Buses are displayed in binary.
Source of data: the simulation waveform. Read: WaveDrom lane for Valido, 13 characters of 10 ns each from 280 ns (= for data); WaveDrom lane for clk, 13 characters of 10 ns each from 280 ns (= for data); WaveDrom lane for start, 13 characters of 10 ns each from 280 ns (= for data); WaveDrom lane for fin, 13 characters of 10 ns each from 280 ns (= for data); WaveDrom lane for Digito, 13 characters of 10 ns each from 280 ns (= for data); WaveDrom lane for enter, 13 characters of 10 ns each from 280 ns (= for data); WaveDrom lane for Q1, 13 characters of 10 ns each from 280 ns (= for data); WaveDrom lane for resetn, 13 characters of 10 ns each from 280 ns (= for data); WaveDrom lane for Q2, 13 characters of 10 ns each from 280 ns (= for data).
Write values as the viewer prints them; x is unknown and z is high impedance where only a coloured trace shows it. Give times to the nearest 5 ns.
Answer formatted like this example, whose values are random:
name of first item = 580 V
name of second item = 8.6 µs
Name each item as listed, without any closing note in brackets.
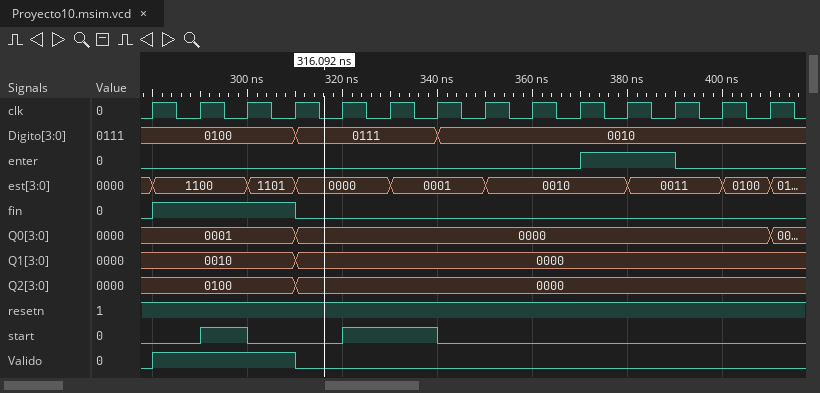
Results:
WaveDrom lane for Valido, 13 characters of 10 ns each from 280 ns = {name: 'Valido', wave: '1..0.........'}
WaveDrom lane for clk, 13 characters of 10 ns each from 280 ns = {name: 'clk', wave: 'p............'}
WaveDrom lane for start, 13 characters of 10 ns each from 280 ns = {name: 'start', wave: '010.1.0......'}
WaveDrom lane for fin, 13 characters of 10 ns each from 280 ns = {name: 'fin', wave: '1..0.........'}
WaveDrom lane for Digito, 13 characters of 10 ns each from 280 ns = {name: 'Digito', wave: '=..=..=......', data: '0100 0111 0010'}
WaveDrom lane for enter, 13 characters of 10 ns each from 280 ns = {name: 'enter', wave: '0........1.0.'}
WaveDrom lane for Q1, 13 characters of 10 ns each from 280 ns = {name: 'Q1', wave: '=..=.........', data: '0010 0000'}
WaveDrom lane for resetn, 13 characters of 10 ns each from 280 ns = {name: 'resetn', wave: '1............'}
WaveDrom lane for Q2, 13 characters of 10 ns each from 280 ns = {name: 'Q2', wave: '=..=.........', data: '0100 0000'}
